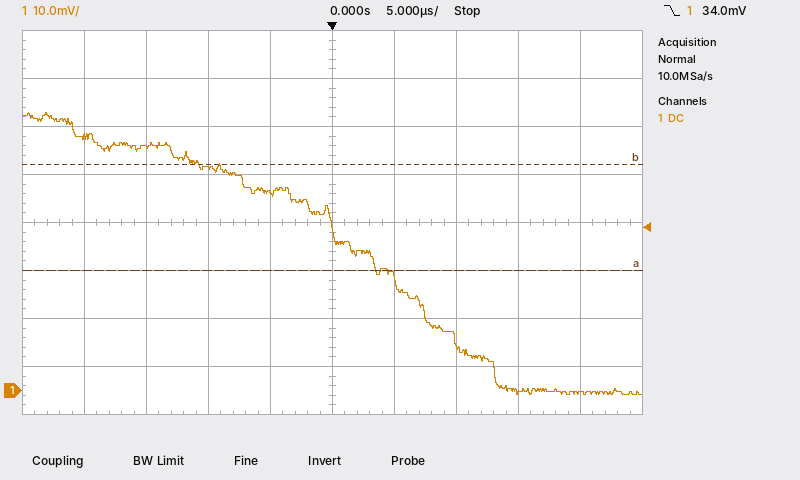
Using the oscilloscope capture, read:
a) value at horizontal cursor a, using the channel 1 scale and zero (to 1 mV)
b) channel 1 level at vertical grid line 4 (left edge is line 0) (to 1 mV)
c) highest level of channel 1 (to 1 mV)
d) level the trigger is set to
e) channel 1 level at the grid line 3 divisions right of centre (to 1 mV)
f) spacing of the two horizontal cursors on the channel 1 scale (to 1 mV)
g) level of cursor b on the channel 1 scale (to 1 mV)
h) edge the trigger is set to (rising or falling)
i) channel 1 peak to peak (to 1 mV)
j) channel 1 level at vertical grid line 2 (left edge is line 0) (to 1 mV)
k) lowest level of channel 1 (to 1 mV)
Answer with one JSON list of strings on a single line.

["25 mV", "41 mV", "58 mV", "34.0 mV", "0 mV", "22 mV", "47 mV", "falling", "59 mV", "51 mV", "-1 mV"]
